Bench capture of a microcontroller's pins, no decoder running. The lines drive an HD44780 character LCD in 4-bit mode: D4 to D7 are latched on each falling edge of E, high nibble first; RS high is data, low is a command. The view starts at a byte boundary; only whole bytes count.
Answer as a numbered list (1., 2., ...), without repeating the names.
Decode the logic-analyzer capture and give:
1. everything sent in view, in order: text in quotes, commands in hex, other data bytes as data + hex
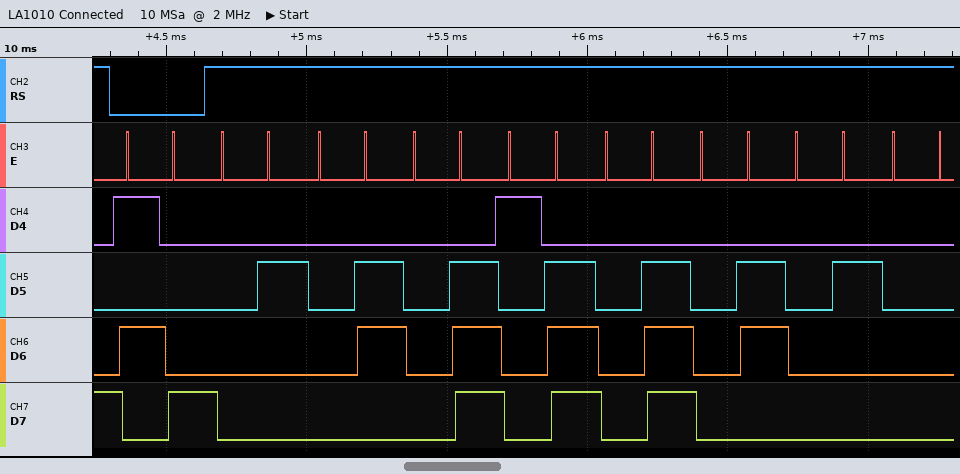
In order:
1. 0x58 data 02 06 0E 1E 0E 06 02 00
